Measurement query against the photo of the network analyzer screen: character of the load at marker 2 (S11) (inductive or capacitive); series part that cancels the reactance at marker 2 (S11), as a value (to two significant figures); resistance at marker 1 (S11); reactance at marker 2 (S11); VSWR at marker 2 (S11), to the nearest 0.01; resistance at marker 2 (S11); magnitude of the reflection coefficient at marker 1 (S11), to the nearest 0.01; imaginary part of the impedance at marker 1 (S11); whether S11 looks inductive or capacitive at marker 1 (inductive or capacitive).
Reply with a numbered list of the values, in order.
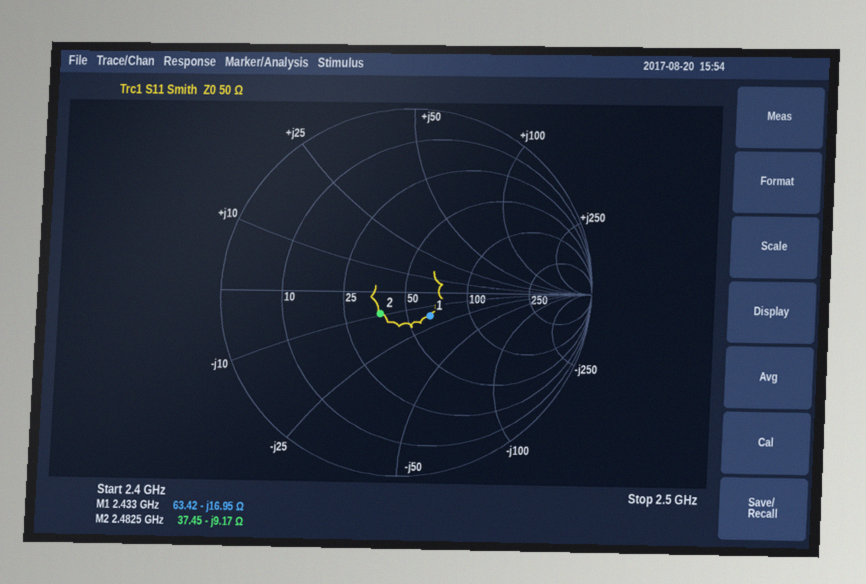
1. capacitive
2. 590 pH
3. 63.42 Ω
4. -9.17 Ω
5. 1.43
6. 37.45 Ω
7. 0.19
8. -16.95 Ω
9. capacitive
